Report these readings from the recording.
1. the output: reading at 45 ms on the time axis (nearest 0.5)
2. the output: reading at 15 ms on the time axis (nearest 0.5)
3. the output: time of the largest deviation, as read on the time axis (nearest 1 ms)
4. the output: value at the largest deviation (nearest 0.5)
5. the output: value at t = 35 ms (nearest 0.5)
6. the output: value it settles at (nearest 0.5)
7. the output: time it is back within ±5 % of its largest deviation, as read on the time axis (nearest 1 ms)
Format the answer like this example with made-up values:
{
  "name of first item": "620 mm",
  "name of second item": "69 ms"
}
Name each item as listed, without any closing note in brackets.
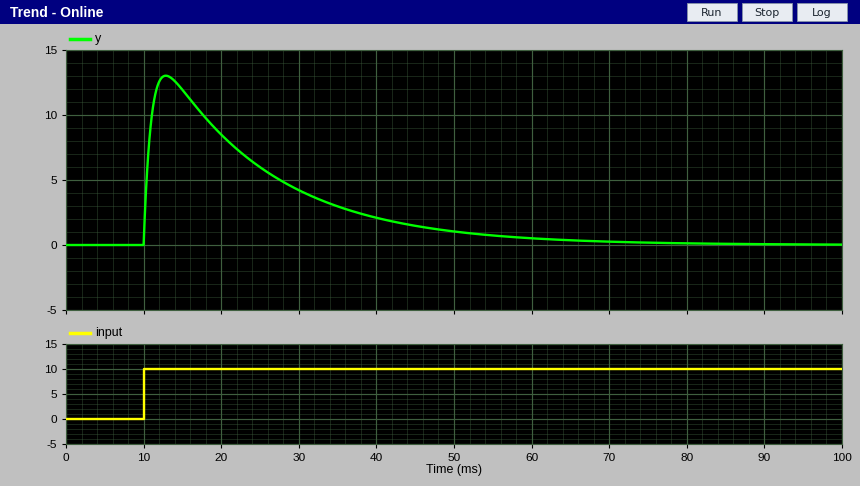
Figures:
{
  "the output: reading at 45 ms on the time axis": "1.5",
  "the output: reading at 15 ms on the time axis": "12.0",
  "the output: time of the largest deviation, as read on the time axis": "13 ms",
  "the output: value at the largest deviation": "13.0",
  "the output: value at t = 35 ms": "3.0",
  "the output: value it settles at": "0.0",
  "the output: time it is back within ±5 % of its largest deviation, as read on the time axis": "57 ms"
}
